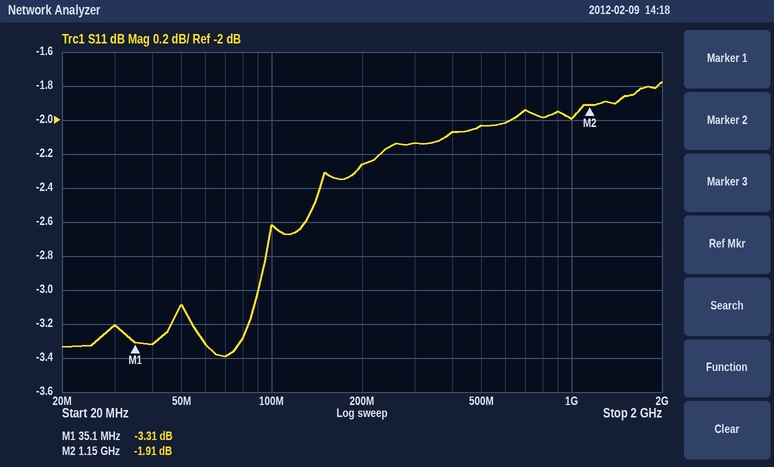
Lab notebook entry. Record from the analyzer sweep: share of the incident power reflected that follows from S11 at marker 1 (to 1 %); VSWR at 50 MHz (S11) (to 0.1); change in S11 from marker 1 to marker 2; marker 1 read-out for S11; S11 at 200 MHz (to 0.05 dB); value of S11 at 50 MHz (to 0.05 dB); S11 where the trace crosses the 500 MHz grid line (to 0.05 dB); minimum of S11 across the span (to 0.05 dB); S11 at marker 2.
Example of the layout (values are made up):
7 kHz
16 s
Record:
47 %
5.7
1.40 dB
-3.31 dB
-2.25 dB
-3.10 dB
-2.05 dB
-3.40 dB
-1.91 dB
